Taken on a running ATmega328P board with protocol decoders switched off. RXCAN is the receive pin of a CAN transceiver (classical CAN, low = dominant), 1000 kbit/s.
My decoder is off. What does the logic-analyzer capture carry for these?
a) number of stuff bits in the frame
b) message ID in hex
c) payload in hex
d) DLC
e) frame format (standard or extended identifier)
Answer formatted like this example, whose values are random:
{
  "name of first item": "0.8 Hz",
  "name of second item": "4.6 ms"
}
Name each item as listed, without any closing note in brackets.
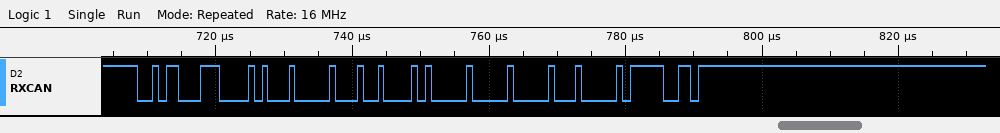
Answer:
{
  "number of stuff bits in the frame": "6",
  "message ID in hex": "0x2C7",
  "payload in hex": "10 09 0A 00 00",
  "DLC": "5",
  "frame format": "standard"
}
